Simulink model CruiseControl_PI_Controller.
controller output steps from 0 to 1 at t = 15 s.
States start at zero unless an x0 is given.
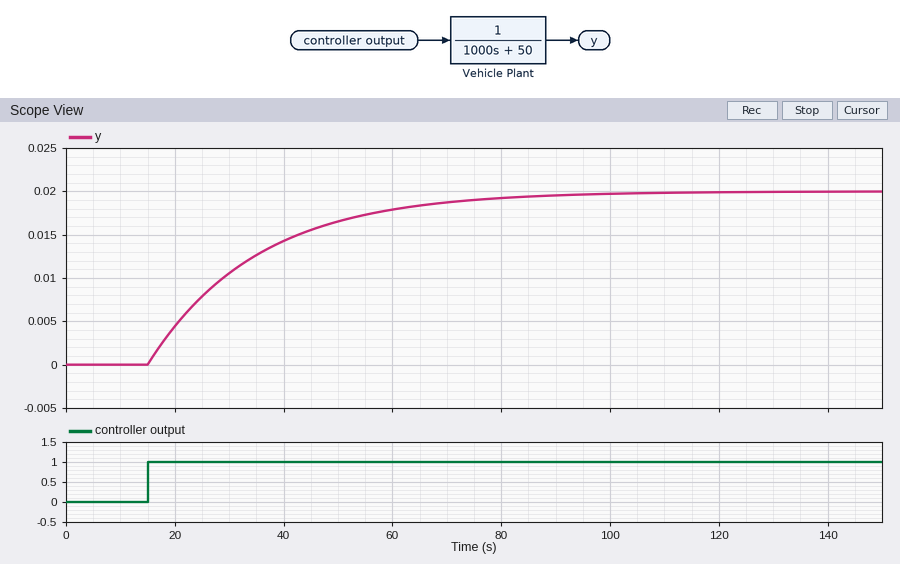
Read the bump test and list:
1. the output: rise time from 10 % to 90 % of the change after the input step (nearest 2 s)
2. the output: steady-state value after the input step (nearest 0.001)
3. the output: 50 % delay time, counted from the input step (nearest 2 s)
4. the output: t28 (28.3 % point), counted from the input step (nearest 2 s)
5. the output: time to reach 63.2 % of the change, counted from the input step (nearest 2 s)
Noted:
44 s
0.020
14 s
6 s
20 s
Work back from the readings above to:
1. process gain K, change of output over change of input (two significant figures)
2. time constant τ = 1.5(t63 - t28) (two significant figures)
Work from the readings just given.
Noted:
0.020
21 s
